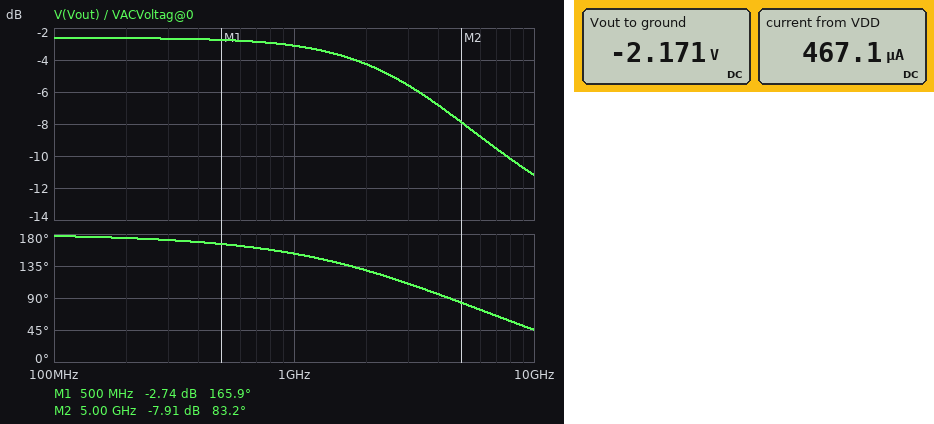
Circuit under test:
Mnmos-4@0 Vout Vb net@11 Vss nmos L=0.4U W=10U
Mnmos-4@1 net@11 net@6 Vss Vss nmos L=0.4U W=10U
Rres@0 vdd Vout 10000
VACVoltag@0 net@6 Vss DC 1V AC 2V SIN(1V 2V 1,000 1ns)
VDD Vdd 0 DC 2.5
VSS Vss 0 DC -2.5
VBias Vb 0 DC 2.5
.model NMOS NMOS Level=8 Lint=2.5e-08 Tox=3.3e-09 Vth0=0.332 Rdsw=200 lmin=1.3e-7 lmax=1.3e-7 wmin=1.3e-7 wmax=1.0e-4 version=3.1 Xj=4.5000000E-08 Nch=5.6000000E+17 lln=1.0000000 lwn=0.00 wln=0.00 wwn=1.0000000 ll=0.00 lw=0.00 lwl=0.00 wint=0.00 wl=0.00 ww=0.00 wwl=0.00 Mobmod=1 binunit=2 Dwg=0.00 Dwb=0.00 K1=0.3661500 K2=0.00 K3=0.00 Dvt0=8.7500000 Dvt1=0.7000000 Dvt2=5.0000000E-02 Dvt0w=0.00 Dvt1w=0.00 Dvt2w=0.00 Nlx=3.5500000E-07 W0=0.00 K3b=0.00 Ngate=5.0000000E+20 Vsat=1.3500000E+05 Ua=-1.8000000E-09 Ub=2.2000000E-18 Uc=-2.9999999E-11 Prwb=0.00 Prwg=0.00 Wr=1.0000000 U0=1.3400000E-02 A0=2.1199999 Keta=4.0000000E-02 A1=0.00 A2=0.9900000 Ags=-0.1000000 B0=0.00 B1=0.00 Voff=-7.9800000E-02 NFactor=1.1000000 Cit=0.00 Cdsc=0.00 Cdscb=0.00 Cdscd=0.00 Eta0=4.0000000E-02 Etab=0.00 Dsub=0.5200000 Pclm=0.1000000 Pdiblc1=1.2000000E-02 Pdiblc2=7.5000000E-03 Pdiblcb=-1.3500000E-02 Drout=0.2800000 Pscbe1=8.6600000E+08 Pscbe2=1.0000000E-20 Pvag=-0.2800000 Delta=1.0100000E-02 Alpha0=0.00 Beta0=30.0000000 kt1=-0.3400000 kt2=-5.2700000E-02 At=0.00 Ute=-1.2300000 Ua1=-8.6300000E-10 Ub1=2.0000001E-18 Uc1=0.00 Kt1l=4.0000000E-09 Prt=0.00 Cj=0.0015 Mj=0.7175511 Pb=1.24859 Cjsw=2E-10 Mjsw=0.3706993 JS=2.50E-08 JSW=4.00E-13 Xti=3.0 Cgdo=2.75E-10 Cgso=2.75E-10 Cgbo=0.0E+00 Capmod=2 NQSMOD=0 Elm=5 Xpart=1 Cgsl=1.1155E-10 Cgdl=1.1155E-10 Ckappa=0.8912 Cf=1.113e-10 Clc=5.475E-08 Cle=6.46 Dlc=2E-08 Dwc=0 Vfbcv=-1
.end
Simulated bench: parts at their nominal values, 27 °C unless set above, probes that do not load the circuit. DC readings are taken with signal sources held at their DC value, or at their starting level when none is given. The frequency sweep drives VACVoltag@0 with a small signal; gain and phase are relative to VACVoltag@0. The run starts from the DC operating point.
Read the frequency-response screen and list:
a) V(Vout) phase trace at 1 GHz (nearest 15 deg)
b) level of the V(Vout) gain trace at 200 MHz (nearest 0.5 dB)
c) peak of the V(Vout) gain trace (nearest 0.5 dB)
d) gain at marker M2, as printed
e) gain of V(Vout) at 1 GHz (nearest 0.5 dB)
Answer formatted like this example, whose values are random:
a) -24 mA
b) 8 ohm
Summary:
a) 150 deg
b) -2.5 dB
c) -2.5 dB
d) -7.91 dB
e) -3.0 dB
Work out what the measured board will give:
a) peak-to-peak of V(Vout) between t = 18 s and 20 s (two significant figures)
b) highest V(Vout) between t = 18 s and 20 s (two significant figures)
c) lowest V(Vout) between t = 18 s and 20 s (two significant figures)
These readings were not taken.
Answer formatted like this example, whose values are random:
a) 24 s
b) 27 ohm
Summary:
a) 4.8 V
b) 2.5 V
c) -2.3 V
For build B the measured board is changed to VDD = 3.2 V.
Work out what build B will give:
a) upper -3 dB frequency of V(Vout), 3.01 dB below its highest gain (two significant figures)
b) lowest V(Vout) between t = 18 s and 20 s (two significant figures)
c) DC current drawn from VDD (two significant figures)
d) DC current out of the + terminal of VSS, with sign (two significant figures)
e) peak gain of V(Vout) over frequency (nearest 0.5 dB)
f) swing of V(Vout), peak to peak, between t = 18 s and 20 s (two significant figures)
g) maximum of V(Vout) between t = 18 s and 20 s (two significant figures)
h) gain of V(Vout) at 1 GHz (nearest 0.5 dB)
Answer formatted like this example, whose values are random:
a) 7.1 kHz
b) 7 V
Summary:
a) 2.2 GHz
b) -2.3 V
c) 530 µA
d) -530 µA
e) 2.0 dB
f) 5.5 V
g) 3.2 V
h) 1.0 dB
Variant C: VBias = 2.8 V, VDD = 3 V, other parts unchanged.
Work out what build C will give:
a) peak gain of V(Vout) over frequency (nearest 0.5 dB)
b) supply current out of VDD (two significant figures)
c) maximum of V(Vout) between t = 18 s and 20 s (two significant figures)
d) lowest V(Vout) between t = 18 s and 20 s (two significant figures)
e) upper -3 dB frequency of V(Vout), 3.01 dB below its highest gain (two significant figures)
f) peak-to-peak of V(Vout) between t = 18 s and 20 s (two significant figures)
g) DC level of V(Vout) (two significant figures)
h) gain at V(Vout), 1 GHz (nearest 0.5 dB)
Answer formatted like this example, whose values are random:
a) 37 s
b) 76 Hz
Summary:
a) 0.5 dB
b) 510 µA
c) 3.0 V
d) -2.3 V
e) 2.5 GHz
f) 5.3 V
g) -2.1 V
h) -0.5 dB
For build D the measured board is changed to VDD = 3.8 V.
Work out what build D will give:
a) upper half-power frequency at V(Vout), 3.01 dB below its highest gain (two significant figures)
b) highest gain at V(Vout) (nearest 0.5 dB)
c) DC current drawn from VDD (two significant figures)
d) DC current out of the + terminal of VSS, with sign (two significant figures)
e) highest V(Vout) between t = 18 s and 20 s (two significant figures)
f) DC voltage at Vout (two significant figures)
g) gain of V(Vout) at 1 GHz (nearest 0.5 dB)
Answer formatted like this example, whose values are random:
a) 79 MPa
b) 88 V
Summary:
a) 1.4 GHz
b) 8.5 dB
c) 580 µA
d) -580 µA
e) 3.8 V
f) -2.0 V
g) 6.5 dB
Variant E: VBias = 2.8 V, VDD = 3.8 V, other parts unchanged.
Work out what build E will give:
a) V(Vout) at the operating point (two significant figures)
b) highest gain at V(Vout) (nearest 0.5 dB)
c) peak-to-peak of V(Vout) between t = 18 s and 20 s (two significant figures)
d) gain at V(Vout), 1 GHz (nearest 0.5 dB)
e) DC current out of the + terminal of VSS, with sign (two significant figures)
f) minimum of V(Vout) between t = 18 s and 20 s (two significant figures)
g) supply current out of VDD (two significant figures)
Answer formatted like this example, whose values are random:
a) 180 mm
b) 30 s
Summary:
a) -2.0 V
b) 8.5 dB
c) 6.0 V
d) 6.5 dB
e) -580 µA
f) -2.2 V
g) 580 µA
